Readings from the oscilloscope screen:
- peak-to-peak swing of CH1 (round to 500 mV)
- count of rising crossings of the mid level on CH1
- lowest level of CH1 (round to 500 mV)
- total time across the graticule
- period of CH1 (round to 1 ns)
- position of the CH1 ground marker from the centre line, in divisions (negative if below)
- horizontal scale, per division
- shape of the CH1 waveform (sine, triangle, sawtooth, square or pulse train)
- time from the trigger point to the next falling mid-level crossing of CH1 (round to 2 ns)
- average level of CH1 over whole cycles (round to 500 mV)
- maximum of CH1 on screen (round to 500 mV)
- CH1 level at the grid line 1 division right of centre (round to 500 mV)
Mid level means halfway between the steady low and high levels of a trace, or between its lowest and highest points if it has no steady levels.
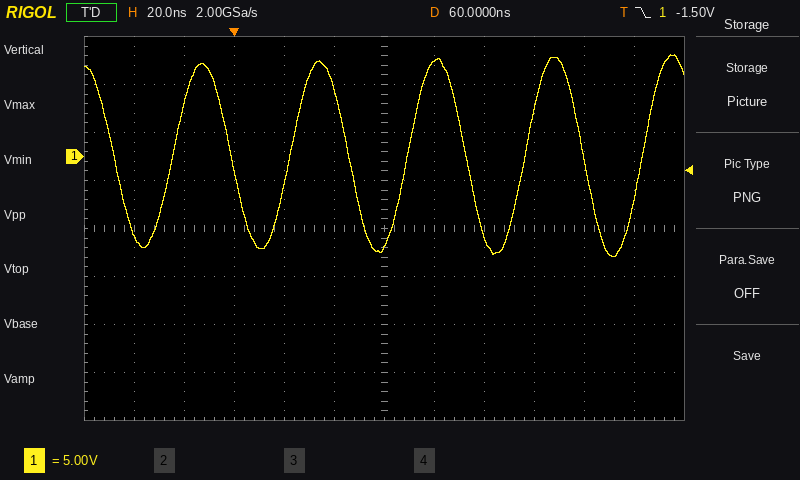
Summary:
21.0 V
5
-10.5 V
240 ns
47 ns
+1.5 div
20 ns
sine
46 ns
0.0 V
10.5 V
10.0 V
